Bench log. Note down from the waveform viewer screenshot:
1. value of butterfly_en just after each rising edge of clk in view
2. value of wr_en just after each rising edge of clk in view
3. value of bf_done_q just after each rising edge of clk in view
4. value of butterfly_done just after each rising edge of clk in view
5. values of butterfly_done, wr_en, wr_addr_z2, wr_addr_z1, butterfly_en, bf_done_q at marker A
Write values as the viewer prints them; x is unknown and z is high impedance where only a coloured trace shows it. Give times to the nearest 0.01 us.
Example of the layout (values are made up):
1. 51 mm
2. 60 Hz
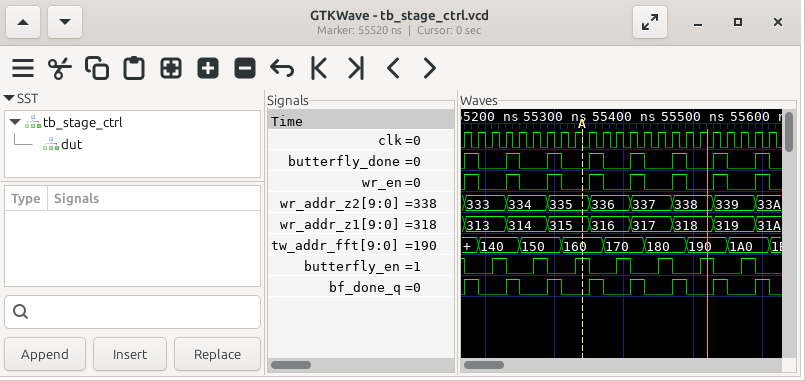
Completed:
1. 0 0 1 0 0 1 0 0 1 0 0 1 0 0 1 0 0 1 0 0 1 0 0
2. 1 0 0 1 0 0 1 0 0 1 0 0 1 0 0 1 0 0 1 0 0 1 0
3. 1 0 0 1 0 0 1 0 0 1 0 0 1 0 0 1 0 0 1 0 0 1 0
4. 1 0 0 1 0 0 1 0 0 1 0 0 1 0 0 1 0 0 1 0 0 1 0
5. butterfly_done=0, wr_en=0, wr_addr_z2=335, wr_addr_z1=315, butterfly_en=1, bf_done_q=0
